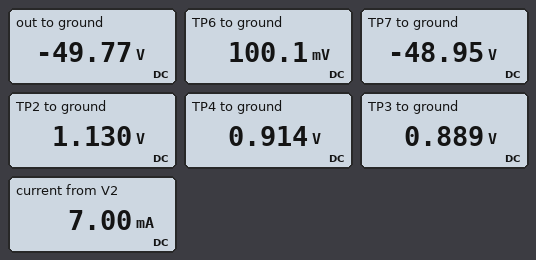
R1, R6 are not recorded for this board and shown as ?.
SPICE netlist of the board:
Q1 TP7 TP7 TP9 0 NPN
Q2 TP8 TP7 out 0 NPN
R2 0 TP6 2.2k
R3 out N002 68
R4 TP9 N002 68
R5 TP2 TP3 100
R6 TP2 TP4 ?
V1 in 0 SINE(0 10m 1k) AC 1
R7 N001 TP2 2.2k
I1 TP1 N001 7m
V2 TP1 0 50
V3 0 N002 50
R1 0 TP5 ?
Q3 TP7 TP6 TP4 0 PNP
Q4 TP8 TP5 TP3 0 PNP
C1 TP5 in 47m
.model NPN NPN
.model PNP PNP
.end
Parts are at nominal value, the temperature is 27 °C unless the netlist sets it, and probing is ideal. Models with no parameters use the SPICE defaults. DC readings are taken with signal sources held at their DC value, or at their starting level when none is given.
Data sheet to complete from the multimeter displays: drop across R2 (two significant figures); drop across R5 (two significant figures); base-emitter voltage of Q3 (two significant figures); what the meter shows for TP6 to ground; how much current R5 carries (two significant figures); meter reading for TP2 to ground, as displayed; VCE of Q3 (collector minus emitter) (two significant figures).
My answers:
100 mV
240 mV
-810 mV
100.1 mV
2.4 mA
1.130 V
-50 V
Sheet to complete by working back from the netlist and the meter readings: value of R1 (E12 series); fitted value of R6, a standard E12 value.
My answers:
3.9 kΩ
47 Ω
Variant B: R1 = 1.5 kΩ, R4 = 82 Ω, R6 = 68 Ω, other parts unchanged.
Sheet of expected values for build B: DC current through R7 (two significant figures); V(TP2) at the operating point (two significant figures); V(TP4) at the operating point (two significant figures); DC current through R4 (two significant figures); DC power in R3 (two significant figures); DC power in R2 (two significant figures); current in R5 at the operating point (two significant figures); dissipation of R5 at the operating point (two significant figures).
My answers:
7.0 mA
1.2 V
890 mV
3.2 mA
950 µW
3.3 µW
3.1 mA
960 µW
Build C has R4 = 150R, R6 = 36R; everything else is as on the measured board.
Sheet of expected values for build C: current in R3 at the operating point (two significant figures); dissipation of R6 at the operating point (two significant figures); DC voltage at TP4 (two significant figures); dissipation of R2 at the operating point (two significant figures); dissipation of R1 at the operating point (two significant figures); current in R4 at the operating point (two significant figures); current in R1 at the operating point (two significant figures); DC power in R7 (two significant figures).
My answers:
4.6 mA
840 µW
920 mV
5.0 µW
1.8 µW
2.3 mA
21 µA
110 mW
